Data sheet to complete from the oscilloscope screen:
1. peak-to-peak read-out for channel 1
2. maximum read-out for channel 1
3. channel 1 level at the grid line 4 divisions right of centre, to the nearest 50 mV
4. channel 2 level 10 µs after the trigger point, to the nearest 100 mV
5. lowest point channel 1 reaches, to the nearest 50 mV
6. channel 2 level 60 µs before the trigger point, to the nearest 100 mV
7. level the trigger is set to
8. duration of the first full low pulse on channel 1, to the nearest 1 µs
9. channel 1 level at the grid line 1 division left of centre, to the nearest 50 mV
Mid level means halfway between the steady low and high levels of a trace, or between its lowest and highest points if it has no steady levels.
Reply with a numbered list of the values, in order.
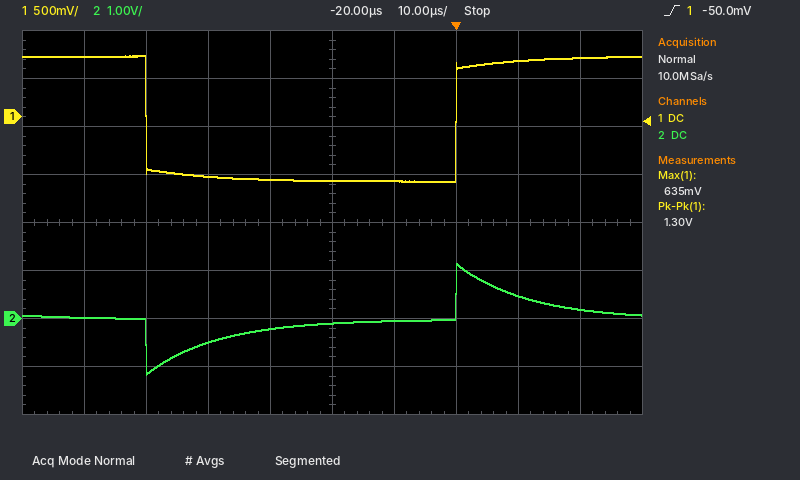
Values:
1. 1.30 V
2. 635 mV
3. 600 mV
4. 500 mV
5. -650 mV
6. 0.0 V
7. -50.0 mV
8. 50 µs
9. -650 mV
